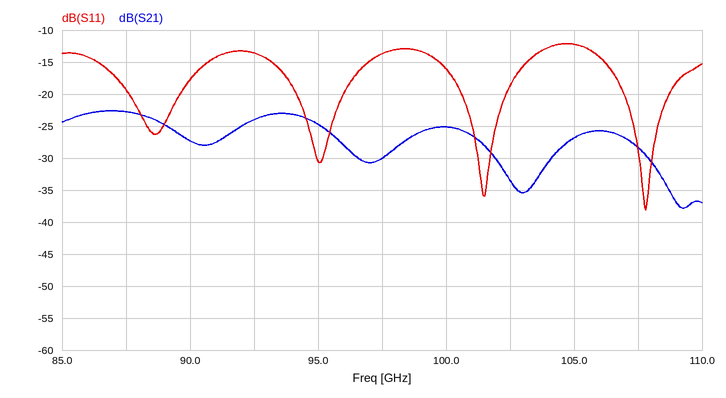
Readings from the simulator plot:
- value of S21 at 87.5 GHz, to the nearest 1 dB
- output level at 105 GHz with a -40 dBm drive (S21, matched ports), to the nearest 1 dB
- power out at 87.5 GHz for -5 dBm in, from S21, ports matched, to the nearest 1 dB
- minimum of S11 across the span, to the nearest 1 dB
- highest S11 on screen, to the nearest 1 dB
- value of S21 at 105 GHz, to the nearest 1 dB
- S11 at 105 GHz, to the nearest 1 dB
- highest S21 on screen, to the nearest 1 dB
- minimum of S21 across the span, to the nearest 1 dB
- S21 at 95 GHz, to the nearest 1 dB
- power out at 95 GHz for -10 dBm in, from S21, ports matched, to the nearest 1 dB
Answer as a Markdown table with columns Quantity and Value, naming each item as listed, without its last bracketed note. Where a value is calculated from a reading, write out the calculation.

| Quantity | Value |
|---|---|
| value of S21 at 87.5 GHz, to the nearest 1 dB | -23 dB |
| output level at 105 GHz with a -40 dBm drive (S21, matched ports), to the nearest 1 dB | -40 dBm + (-27 dB) = -67 dBm |
| power out at 87.5 GHz for -5 dBm in, from S21, ports matched, to the nearest 1 dB | -5 dBm + (-23 dB) = -28 dBm |
| minimum of S11 across the span, to the nearest 1 dB | -38 dB |
| highest S11 on screen, to the nearest 1 dB | -12 dB |
| value of S21 at 105 GHz, to the nearest 1 dB | -27 dB |
| S11 at 105 GHz, to the nearest 1 dB | -12 dB |
| highest S21 on screen, to the nearest 1 dB | -23 dB |
| minimum of S21 across the span, to the nearest 1 dB | -38 dB |
| S21 at 95 GHz, to the nearest 1 dB | -25 dB |
| power out at 95 GHz for -10 dBm in, from S21, ports matched, to the nearest 1 dB | -10 dBm + (-25 dB) = -35 dBm |
